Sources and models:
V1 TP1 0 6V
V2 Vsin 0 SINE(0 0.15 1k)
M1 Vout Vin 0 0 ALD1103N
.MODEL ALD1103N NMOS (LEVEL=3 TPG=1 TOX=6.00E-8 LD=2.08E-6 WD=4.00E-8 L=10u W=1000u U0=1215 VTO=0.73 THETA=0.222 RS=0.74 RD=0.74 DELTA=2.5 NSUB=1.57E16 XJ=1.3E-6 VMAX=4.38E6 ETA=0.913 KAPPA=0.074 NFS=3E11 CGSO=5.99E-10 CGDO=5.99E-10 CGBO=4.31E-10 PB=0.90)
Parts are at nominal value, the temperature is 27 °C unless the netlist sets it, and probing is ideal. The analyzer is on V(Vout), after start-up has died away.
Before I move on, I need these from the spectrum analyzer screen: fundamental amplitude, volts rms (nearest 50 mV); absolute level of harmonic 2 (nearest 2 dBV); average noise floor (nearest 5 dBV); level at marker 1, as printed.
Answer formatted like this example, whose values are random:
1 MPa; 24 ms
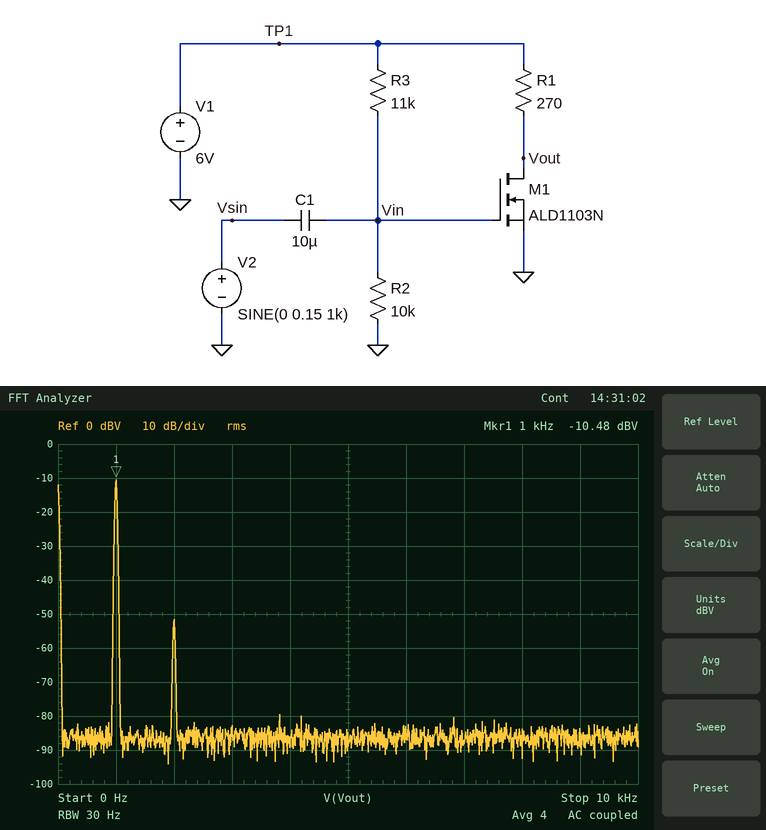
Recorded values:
300 mV; -52 dBV; -85 dBV; -10.48 dBV
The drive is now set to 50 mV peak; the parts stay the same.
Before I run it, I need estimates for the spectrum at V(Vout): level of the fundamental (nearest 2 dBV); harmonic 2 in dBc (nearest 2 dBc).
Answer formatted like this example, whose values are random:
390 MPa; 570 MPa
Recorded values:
-20 dBV; -50 dBc
